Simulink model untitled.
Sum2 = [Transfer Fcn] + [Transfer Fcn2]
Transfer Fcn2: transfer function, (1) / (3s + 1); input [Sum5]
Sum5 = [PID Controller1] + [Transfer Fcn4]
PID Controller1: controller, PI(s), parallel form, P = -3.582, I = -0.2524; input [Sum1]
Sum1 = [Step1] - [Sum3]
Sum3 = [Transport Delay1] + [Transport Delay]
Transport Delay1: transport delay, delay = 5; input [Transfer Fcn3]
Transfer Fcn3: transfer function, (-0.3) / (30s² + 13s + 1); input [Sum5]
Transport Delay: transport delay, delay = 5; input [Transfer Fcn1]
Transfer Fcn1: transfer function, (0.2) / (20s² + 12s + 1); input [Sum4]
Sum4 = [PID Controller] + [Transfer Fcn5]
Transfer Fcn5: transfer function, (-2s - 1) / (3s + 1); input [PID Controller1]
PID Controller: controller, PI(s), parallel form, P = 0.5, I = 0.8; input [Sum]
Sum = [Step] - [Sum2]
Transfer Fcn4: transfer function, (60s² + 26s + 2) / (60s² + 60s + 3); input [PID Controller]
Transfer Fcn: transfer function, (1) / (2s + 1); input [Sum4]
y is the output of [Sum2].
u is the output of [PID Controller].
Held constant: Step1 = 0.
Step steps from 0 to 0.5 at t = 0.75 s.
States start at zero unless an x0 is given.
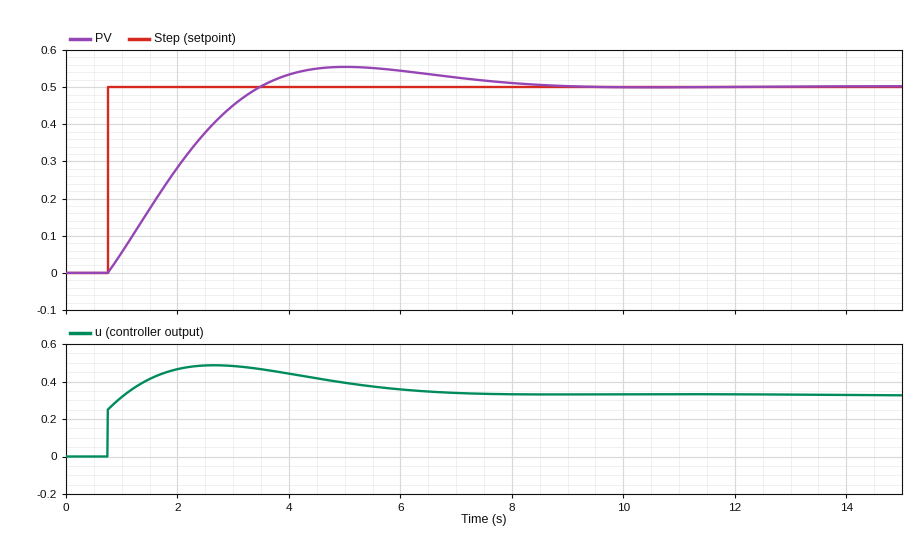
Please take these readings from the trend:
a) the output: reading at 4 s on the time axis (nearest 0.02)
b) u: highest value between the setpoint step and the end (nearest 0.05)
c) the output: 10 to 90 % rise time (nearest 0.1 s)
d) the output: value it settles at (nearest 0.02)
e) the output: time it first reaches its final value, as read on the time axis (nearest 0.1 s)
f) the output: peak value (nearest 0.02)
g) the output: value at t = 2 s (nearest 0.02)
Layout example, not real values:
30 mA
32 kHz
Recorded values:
0.54
0.50
2.0 s
0.50
3.5 s
0.56
0.28
